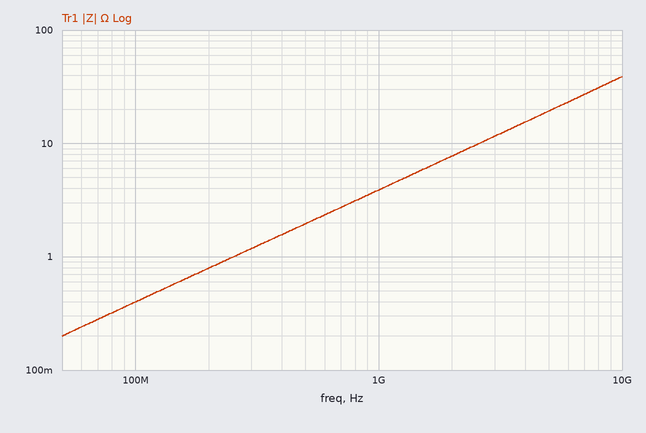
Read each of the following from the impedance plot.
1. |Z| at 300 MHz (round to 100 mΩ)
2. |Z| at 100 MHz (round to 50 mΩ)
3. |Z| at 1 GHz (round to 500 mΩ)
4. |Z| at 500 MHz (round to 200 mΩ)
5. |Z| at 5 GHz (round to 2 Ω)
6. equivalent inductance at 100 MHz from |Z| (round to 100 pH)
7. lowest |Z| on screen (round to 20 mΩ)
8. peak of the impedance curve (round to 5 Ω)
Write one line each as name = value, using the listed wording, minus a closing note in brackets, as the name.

|Z| at 300 MHz = 1.2 Ω
|Z| at 100 MHz = 400 mΩ
|Z| at 1 GHz = 4.0 Ω
|Z| at 500 MHz = 2.0 Ω
|Z| at 5 GHz = 20 Ω
equivalent inductance at 100 MHz from |Z| = 600 pH
lowest |Z| on screen = 200 mΩ
peak of the impedance curve = 40 Ω
